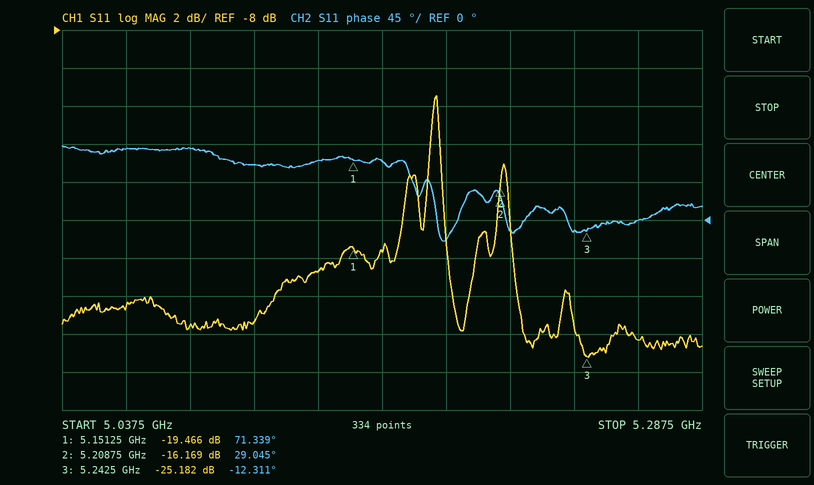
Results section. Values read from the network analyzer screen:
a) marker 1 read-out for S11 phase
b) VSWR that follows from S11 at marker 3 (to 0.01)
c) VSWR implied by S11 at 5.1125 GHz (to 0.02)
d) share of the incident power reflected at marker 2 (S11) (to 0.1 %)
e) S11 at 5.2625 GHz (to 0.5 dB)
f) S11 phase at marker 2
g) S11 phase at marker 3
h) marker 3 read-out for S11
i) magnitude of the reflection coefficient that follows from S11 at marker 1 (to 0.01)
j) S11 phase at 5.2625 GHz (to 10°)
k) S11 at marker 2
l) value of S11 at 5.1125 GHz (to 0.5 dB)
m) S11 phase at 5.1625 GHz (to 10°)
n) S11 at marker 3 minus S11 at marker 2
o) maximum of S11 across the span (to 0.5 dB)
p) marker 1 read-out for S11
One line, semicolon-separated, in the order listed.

71.339°; 1.12; 1.14; 2.4 %; -24.5 dB; 29.045°; -12.311°; -25.182 dB; 0.11; 0°; -16.169 dB; -23.5 dB; 70°; -9.013 dB; -11.5 dB; -19.466 dB
